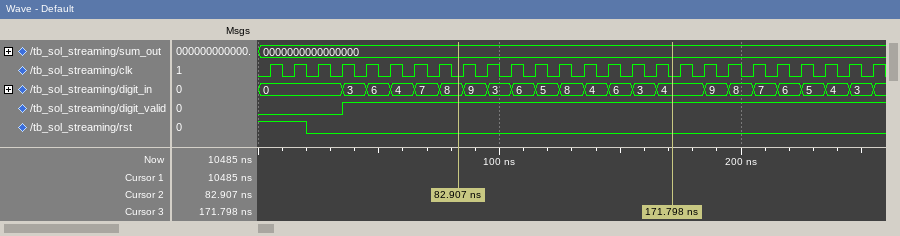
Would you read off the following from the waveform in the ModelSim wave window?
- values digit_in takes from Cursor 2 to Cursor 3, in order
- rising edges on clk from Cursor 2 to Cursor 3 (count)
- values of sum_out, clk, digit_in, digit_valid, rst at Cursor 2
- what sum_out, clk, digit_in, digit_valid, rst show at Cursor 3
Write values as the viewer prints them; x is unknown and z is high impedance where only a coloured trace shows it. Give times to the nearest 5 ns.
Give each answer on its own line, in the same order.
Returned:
8, 9, 3, 6, 5, 8, 4, 6, 3, 4
9
sum_out=0000000000000000, clk=0, digit_in=8, digit_valid=1, rst=0
sum_out=0000000000000000, clk=0, digit_in=4, digit_valid=1, rst=0
